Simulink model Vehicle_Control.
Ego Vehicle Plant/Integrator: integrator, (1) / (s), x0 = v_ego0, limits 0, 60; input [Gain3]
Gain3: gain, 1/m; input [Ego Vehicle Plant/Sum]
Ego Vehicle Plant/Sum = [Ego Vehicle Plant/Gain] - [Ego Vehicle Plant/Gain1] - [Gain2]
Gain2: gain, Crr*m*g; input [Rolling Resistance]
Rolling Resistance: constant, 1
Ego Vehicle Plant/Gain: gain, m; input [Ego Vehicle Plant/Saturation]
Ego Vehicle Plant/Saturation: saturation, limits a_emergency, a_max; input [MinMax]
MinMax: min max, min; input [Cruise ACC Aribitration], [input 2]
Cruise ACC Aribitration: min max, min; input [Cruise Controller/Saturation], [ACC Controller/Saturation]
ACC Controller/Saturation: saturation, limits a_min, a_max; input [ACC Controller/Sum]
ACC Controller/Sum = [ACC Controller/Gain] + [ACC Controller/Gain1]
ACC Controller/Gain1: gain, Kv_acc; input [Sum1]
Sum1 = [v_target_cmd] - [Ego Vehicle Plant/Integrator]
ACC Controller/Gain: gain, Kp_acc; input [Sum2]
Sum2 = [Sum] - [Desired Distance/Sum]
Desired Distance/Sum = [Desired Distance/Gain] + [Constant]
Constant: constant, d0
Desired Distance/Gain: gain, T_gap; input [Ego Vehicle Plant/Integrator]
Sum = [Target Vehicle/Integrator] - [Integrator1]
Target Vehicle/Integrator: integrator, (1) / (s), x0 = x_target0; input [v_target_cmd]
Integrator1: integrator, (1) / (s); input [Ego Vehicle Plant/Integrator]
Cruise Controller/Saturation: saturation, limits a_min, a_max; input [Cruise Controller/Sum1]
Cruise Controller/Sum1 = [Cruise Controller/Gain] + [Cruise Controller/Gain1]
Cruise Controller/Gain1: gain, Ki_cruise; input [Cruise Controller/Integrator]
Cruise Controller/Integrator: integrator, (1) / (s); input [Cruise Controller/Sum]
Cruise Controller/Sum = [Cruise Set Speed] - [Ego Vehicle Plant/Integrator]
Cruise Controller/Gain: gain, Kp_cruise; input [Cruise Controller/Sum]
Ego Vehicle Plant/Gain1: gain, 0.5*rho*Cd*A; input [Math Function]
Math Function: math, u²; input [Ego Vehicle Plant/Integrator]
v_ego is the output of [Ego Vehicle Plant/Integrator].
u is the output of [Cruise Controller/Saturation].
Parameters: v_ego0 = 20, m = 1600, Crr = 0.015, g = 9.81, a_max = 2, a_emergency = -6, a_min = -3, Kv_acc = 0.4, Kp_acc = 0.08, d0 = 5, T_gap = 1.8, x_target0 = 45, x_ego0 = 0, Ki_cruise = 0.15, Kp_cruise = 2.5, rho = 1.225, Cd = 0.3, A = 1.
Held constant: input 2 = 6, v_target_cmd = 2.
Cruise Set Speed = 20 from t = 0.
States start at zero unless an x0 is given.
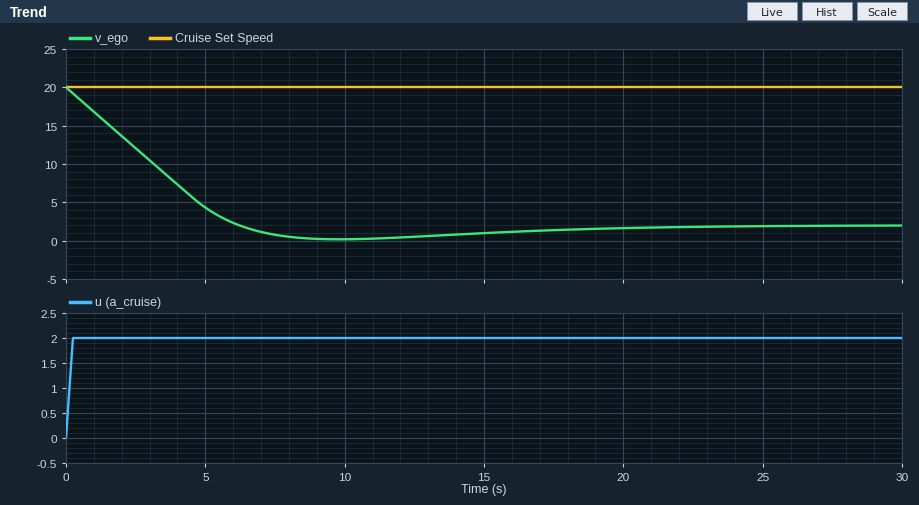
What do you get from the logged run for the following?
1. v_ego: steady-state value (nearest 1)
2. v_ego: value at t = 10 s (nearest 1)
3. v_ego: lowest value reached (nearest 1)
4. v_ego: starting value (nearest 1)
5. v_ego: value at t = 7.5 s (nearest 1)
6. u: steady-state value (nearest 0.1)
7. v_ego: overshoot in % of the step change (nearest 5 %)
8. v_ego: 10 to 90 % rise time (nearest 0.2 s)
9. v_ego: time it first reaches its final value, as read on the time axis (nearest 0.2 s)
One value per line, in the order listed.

2
0
0
20
1
2.0
10 %
4.6 s
6.2 s
